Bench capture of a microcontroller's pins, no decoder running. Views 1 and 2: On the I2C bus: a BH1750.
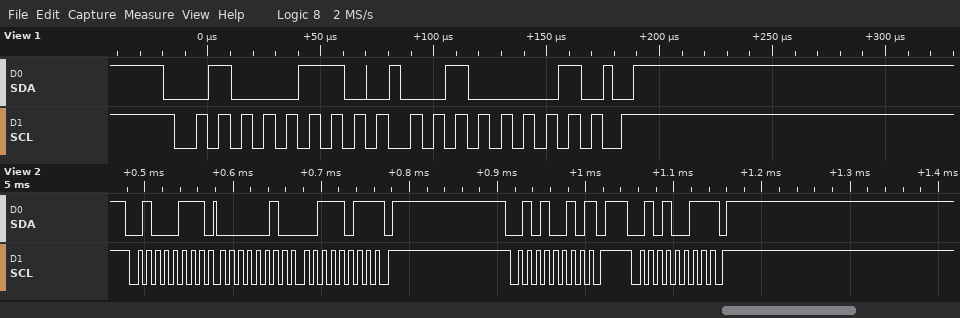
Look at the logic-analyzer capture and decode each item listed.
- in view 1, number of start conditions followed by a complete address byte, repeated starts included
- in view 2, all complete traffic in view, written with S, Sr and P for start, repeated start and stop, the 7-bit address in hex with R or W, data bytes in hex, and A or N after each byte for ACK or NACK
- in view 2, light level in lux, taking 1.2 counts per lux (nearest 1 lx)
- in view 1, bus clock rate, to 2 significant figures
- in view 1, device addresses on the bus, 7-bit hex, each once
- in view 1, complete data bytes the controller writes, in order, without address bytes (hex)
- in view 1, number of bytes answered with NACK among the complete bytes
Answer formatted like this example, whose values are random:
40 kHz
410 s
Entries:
1
S 23R A 02 A 3B N P S 29W N P S 29R N P
476 lx
100 kHz
0x23
21
0
